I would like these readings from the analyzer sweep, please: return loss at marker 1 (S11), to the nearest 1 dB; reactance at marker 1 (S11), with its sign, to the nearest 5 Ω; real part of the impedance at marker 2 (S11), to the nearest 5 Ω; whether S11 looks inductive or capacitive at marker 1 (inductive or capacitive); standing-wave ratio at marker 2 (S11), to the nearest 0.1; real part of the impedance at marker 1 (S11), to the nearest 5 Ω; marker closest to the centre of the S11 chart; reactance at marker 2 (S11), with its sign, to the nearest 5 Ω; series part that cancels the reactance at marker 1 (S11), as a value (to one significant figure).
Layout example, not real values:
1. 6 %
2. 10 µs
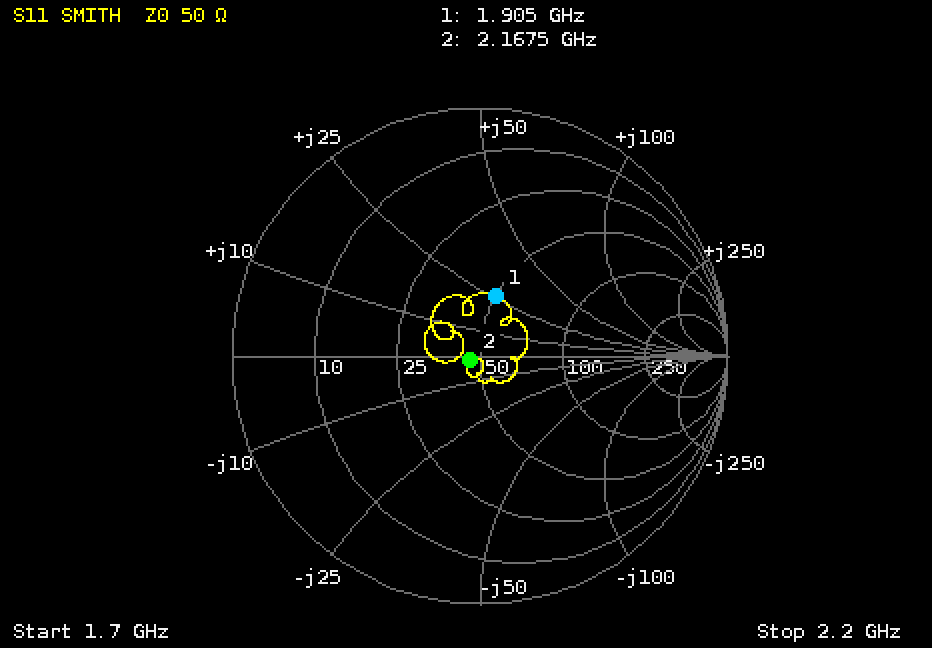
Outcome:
1. 12 dB
2. +25 Ω
3. 45 Ω
4. inductive
5. 1.1
6. 50 Ω
7. marker 2
8. 0 Ω
9. 3 pF
